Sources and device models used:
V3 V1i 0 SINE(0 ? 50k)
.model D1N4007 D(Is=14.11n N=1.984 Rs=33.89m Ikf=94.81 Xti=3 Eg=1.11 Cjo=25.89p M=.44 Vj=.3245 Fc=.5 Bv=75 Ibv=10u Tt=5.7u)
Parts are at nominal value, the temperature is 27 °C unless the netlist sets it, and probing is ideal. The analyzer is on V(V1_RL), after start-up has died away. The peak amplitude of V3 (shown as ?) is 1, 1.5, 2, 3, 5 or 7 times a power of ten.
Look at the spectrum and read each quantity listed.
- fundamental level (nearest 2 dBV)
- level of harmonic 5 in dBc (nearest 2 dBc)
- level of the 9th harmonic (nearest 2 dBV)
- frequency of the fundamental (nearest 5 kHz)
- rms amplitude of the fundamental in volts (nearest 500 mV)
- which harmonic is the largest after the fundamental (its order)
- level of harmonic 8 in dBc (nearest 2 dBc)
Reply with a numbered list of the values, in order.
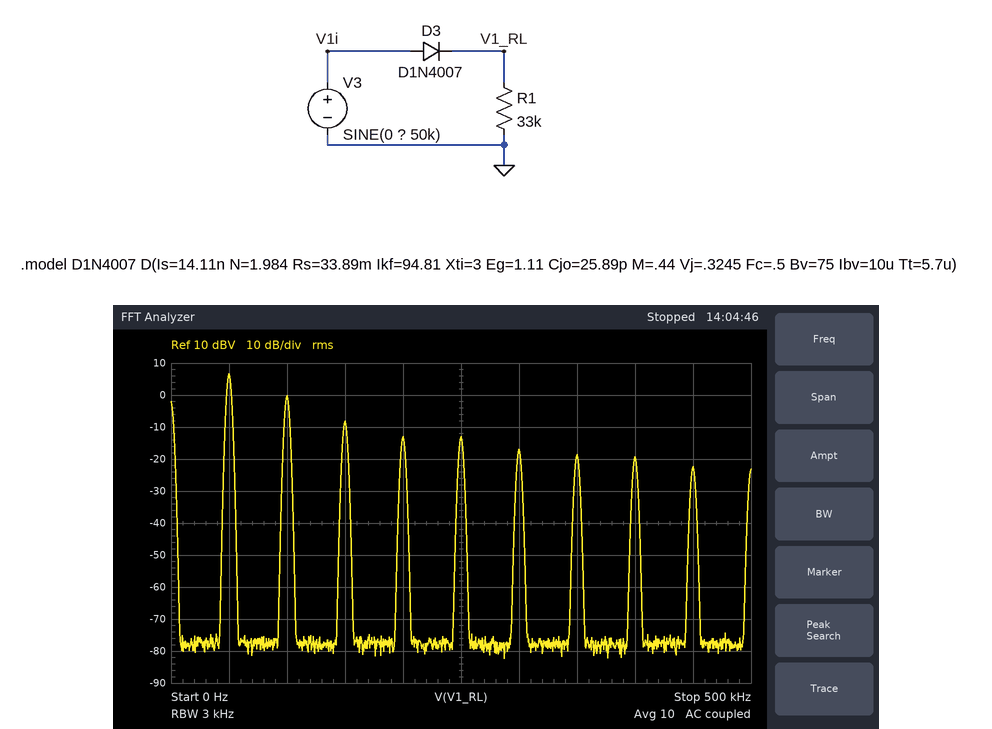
1. 6 dBV
2. -20 dBc
3. -22 dBV
4. 50 kHz
5. 2.0 V
6. 2
7. -26 dBc
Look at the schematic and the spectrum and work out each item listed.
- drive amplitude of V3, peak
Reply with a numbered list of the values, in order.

1. 5 V
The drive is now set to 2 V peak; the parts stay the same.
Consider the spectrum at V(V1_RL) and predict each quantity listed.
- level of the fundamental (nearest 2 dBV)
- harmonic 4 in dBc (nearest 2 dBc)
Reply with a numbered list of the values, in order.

1. -2 dBV
2. -18 dBc
